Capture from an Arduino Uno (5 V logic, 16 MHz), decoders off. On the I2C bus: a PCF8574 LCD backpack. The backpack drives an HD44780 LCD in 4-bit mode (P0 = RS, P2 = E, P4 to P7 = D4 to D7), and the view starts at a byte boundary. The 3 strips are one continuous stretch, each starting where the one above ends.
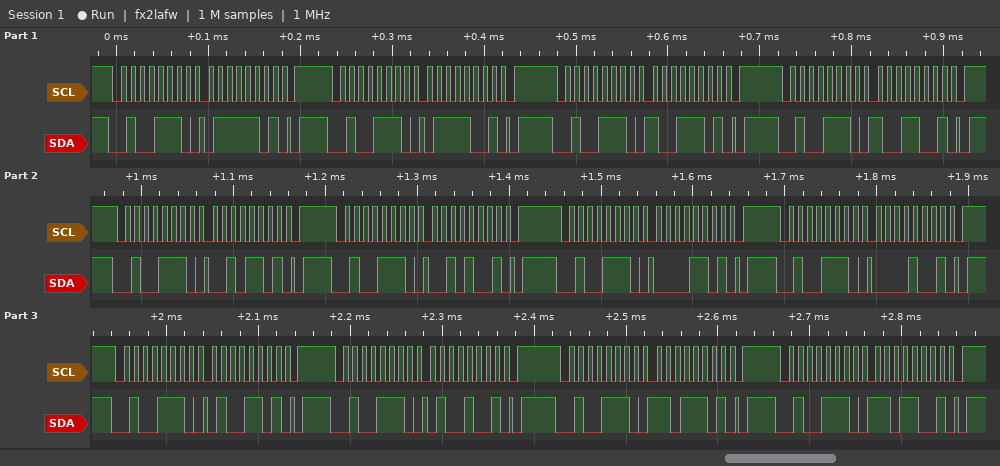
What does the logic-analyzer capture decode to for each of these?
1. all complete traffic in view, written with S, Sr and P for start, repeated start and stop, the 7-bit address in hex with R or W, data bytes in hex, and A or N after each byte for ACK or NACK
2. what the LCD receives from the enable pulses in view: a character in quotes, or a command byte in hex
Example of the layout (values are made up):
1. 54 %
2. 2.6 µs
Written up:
1. S 27W A 7D A P S 27W A 79 A P S 27W A 9D A P S 27W A 99 A P S 27W A 2D A P S 27W A 29 A P S 27W A 0D A P S 27W A 09 A P S 27W A 4D A P S 27W A 49 A P S 27W A DD A P S 27W A D9 A P
2. 'y' ' ' 'M'
